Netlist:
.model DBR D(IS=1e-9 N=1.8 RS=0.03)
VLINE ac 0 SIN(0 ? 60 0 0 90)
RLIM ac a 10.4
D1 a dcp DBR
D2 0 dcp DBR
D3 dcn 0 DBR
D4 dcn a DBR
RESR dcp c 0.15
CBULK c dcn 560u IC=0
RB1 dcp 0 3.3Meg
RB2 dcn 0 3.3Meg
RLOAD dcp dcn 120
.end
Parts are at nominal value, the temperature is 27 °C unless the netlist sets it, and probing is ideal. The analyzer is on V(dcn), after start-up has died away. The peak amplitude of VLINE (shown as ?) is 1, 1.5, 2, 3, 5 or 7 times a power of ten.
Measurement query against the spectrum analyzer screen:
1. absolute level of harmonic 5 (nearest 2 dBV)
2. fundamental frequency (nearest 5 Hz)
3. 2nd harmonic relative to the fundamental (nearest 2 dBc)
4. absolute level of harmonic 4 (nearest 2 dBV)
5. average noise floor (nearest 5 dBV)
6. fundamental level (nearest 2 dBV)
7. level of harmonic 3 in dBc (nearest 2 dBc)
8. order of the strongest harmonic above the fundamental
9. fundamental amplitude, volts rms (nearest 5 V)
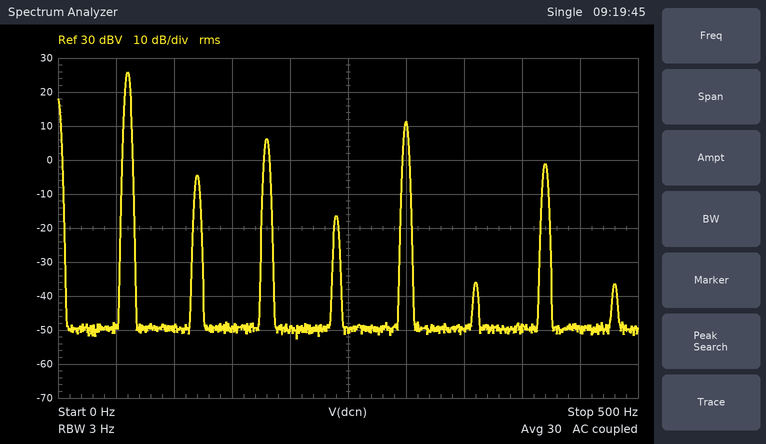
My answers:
12 dBV
60 Hz
-30 dBc
-16 dBV
-50 dBV
26 dBV
-20 dBc
5
20 V
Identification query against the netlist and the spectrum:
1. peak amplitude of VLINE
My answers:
70 V
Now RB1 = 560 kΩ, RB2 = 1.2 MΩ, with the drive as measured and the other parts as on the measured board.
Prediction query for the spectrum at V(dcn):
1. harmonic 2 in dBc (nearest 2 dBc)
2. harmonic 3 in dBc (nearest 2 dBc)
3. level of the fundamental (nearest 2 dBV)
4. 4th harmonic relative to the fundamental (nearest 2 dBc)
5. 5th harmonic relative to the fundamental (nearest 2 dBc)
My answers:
-16 dBc
-22 dBc
26 dBV
-20 dBc
-16 dBc
